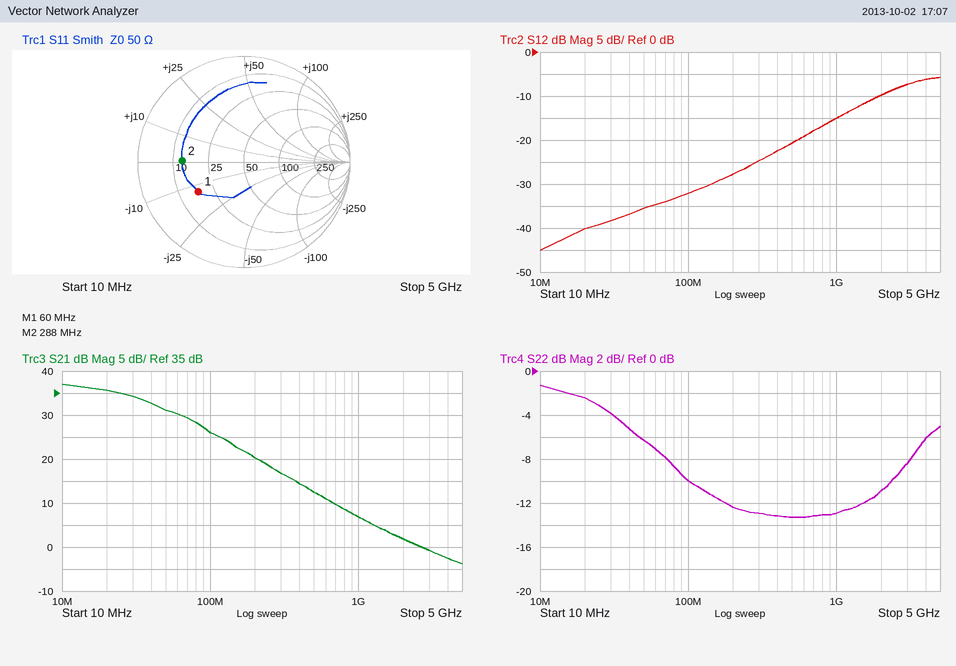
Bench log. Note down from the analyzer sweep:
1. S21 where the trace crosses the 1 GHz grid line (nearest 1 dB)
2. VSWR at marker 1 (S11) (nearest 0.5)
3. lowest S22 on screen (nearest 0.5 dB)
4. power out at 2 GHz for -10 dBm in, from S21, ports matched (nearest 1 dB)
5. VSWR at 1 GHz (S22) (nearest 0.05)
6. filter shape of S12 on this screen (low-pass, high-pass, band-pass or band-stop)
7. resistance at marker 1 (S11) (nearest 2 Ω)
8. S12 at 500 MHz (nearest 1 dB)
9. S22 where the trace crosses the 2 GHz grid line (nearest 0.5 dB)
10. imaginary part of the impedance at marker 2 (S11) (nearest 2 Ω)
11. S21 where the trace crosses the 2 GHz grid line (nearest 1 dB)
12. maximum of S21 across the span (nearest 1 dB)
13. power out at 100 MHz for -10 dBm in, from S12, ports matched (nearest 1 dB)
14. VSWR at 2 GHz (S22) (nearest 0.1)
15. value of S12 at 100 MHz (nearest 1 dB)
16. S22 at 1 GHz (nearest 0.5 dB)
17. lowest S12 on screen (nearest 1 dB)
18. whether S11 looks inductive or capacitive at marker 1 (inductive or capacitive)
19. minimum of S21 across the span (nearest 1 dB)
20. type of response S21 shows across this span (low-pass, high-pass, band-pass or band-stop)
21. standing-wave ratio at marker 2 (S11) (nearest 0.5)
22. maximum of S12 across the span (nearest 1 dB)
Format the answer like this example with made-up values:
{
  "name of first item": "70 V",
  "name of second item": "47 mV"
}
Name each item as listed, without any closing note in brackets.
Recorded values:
{
  "S21 where the trace crosses the 1 GHz grid line": "7 dB",
  "VSWR at marker 1 (S11)": "3.0",
  "lowest S22 on screen": "-13.5 dB",
  "power out at 2 GHz for -10 dBm in, from S21, ports matched": "-8 dBm",
  "VSWR at 1 GHz (S22)": "1.60",
  "filter shape of S12 on this screen": "high-pass",
  "resistance at marker 1 (S11)": "18 Ω",
  "S12 at 500 MHz": "-21 dB",
  "S22 where the trace crosses the 2 GHz grid line": "-11.0 dB",
  "imaginary part of the impedance at marker 2 (S11)": "0 Ω",
  "S21 where the trace crosses the 2 GHz grid line": "2 dB",
  "maximum of S21 across the span": "37 dB",
  "power out at 100 MHz for -10 dBm in, from S12, ports matched": "-42 dBm",
  "VSWR at 2 GHz (S22)": "1.8",
  "value of S12 at 100 MHz": "-32 dB",
  "S22 at 1 GHz": "-13.0 dB",
  "lowest S12 on screen": "-45 dB",
  "whether S11 looks inductive or capacitive at marker 1": "capacitive",
  "minimum of S21 across the span": "-4 dB",
  "type of response S21 shows across this span": "low-pass",
  "standing-wave ratio at marker 2 (S11)": "4.0",
  "maximum of S12 across the span": "-6 dB"
}
